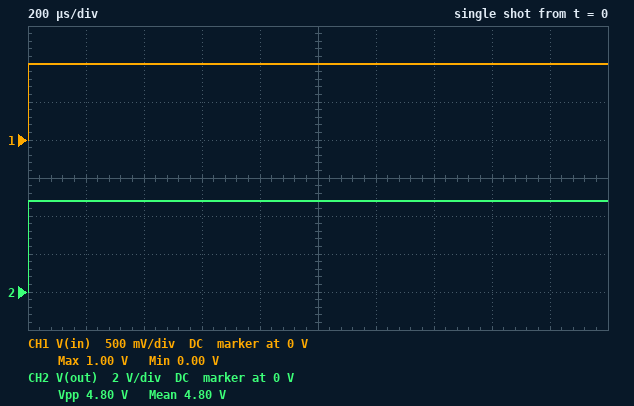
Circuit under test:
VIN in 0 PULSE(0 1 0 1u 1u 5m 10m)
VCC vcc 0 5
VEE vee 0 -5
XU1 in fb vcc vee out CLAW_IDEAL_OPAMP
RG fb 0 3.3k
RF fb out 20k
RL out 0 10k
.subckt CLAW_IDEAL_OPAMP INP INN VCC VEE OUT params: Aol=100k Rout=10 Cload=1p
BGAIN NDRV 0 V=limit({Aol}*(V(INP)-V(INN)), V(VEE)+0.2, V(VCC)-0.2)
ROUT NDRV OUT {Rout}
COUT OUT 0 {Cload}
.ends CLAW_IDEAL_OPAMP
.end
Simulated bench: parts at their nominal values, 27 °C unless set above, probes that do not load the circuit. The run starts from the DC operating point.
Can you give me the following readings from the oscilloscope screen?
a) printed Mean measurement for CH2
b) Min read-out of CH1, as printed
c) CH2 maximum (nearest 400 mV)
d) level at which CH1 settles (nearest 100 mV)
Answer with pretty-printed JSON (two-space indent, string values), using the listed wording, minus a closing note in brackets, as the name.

{
  "printed Mean measurement for CH2": "4.80 V",
  "Min read-out of CH1, as printed": "0.00 V",
  "CH2 maximum": "4.8 V",
  "level at which CH1 settles": "1.0 V"
}
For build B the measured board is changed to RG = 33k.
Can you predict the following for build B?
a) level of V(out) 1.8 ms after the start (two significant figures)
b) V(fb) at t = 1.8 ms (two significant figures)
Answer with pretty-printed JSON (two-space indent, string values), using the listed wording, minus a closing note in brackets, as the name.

{
  "level of V(out) 1.8 ms after the start": "1.6 V",
  "V(fb) at t = 1.8 ms": "1.0 V"
}
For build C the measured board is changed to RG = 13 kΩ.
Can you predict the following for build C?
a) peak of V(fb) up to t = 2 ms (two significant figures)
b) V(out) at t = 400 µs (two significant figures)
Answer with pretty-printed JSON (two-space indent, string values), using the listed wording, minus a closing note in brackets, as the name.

{
  "peak of V(fb) up to t = 2 ms": "1.0 V",
  "V(out) at t = 400 µs": "2.5 V"
}
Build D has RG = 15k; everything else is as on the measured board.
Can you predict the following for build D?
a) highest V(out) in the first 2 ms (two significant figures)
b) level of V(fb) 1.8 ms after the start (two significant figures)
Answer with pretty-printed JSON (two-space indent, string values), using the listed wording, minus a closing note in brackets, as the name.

{
  "highest V(out) in the first 2 ms": "2.3 V",
  "level of V(fb) 1.8 ms after the start": "1.0 V"
}
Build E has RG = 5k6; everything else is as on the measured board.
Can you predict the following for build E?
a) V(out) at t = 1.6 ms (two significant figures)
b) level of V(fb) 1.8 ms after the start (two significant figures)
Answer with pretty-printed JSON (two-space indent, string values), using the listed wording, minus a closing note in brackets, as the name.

{
  "V(out) at t = 1.6 ms": "4.6 V",
  "level of V(fb) 1.8 ms after the start": "1.0 V"
}
